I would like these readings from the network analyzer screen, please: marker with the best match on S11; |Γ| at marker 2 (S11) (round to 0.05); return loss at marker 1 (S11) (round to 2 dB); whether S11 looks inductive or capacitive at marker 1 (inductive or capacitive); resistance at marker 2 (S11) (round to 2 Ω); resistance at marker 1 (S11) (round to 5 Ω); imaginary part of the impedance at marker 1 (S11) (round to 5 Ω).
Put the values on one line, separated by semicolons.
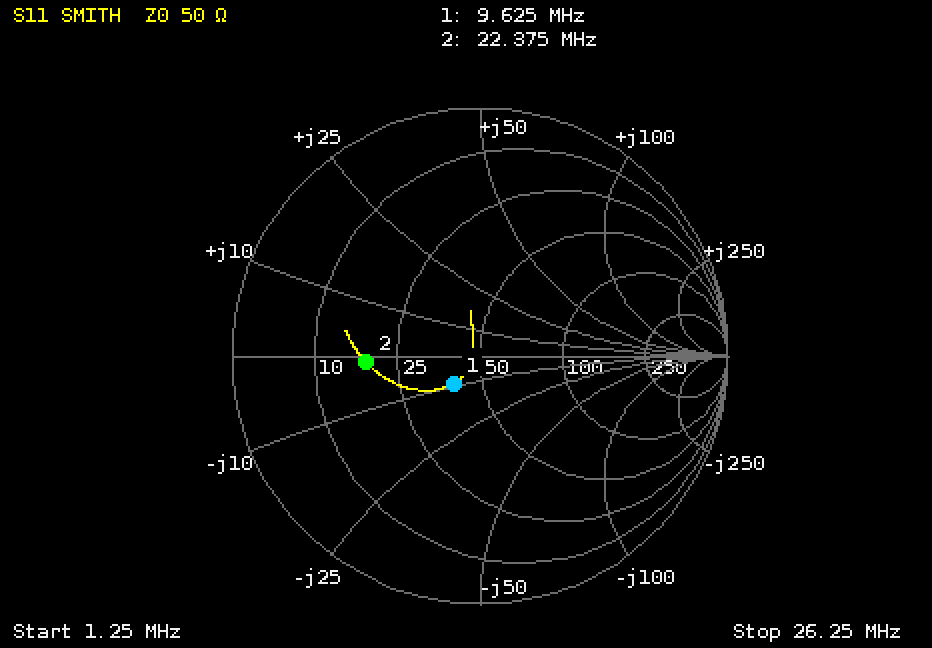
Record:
marker 1; 0.45; 16 dB; capacitive; 18 Ω; 40 Ω; -10 Ω
